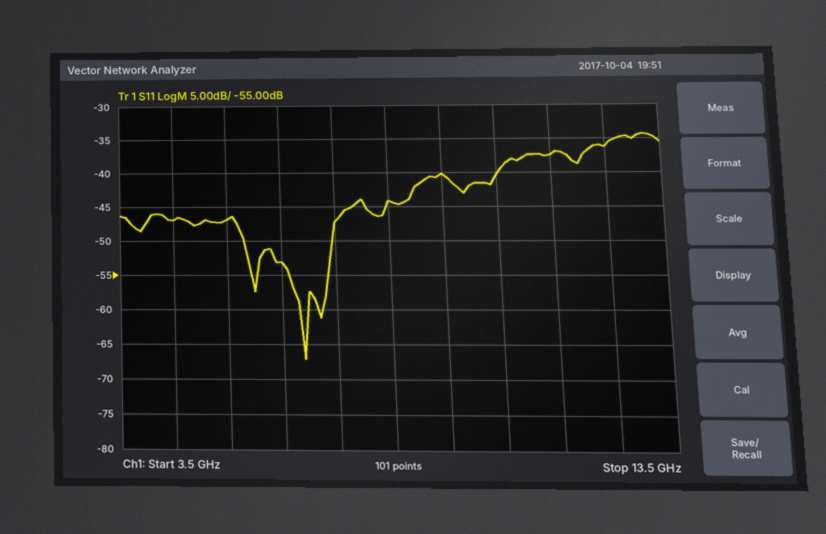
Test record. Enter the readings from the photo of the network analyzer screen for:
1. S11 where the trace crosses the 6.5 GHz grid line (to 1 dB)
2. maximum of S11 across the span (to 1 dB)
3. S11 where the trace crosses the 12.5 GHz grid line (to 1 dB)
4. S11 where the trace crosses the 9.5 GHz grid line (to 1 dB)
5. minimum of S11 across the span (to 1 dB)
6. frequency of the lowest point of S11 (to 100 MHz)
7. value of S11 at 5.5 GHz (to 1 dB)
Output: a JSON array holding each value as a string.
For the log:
["-53 dB", "-34 dB", "-36 dB", "-40 dB", "-67 dB", "6.9 GHz", "-47 dB"]
